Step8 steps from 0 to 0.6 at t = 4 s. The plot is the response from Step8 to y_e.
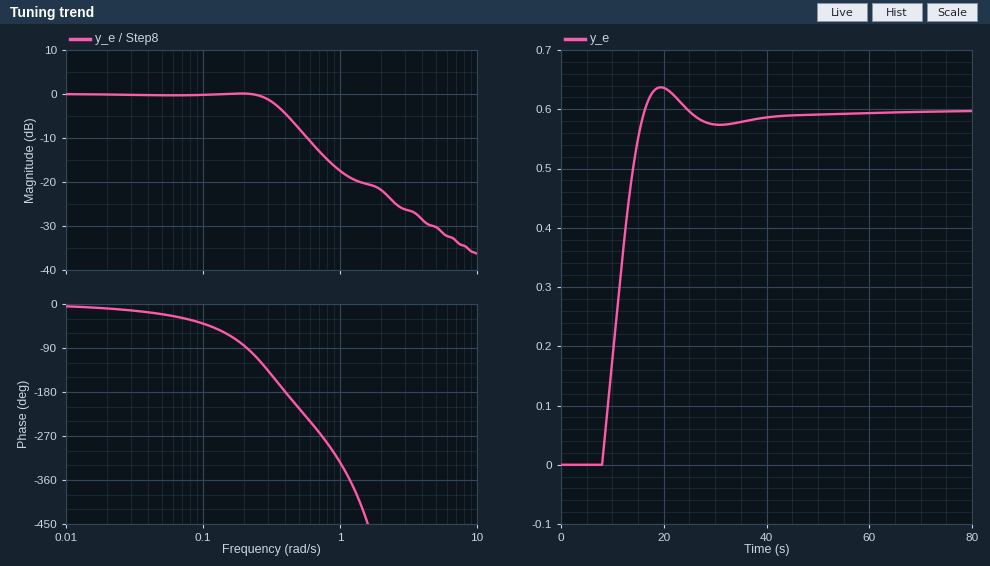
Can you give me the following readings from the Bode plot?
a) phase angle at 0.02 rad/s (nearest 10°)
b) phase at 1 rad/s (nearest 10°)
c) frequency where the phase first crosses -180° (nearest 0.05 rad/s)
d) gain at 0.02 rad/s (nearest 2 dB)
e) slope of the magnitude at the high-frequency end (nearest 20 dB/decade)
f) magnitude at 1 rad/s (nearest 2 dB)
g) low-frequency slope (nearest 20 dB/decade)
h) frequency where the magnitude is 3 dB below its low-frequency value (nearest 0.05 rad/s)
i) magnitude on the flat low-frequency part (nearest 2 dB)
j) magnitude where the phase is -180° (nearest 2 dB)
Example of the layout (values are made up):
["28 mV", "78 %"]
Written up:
["-10°", "-320°", "0.40 rad/s", "0 dB", "-20 dB/decade", "-18 dB", "0 dB/decade", "0.35 rad/s", "0 dB", "-4 dB"]
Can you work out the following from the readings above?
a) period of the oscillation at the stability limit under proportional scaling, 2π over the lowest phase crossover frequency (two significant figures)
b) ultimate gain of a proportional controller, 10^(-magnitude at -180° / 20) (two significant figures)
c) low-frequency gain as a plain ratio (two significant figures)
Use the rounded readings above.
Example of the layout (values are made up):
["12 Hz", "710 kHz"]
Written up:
["16 s", "1.6", "1.0"]
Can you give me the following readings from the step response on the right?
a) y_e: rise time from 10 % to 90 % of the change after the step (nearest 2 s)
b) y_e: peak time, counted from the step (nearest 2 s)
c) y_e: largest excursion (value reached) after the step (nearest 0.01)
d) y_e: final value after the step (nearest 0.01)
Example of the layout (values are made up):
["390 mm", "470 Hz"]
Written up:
["6 s", "16 s", "0.64", "0.60"]
